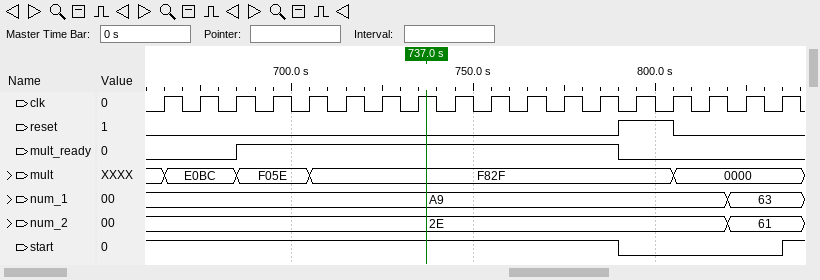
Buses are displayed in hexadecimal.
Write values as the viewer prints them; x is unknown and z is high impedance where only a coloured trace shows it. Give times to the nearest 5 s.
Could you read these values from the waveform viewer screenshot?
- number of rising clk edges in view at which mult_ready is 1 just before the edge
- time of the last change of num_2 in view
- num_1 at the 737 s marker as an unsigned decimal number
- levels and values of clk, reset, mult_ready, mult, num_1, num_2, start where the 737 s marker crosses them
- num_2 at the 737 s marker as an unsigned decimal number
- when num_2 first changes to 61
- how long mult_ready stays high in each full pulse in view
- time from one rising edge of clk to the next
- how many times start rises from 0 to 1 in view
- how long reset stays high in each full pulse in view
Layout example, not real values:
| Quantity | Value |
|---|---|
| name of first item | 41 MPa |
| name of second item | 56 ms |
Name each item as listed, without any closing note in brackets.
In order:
| Quantity | Value |
|---|---|
| number of rising clk edges in view at which mult_ready is 1 just before the edge | 10 |
| time of the last change of num_2 in view | 820 s |
| num_1 at the 737 s marker as an unsigned decimal number | 169 |
| levels and values of clk, reset, mult_ready, mult, num_1, num_2, start where the 737 s marker crosses them | clk=1, reset=0, mult_ready=1, mult=F82F, num_1=A9, num_2=2E, start=1 |
| num_2 at the 737 s marker as an unsigned decimal number | 46 |
| when num_2 first changes to 61 | 820 s |
| how long mult_ready stays high in each full pulse in view | 105 s |
| time from one rising edge of clk to the next | 10 s |
| how many times start rises from 0 to 1 in view | 1 |
| how long reset stays high in each full pulse in view | 15 s |
